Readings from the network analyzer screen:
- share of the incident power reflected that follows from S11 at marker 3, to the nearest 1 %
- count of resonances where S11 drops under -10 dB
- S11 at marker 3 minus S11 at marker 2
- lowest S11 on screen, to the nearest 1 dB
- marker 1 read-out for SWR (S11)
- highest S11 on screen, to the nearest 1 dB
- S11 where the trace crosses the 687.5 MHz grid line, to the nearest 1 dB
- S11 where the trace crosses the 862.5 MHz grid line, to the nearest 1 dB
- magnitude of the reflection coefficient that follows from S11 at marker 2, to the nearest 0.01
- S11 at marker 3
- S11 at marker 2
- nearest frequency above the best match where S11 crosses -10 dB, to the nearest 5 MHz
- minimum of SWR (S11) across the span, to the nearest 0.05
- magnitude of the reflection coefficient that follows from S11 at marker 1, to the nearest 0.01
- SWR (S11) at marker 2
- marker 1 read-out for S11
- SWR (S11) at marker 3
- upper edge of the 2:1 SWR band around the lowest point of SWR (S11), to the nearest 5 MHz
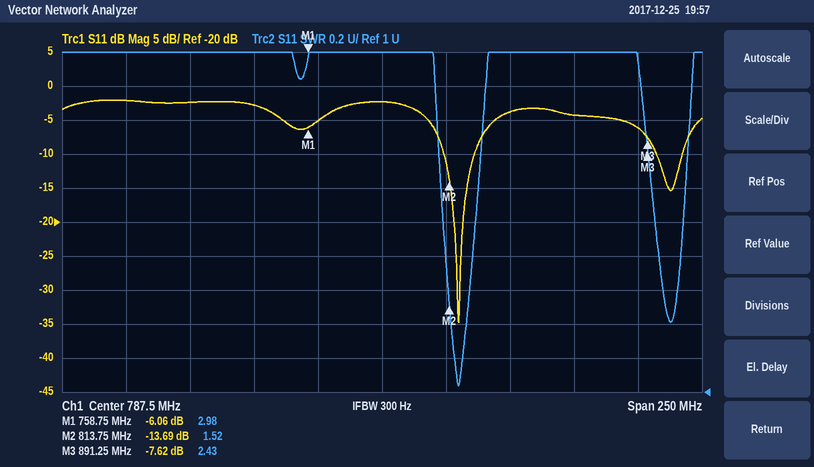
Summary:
17 %
2
6.07 dB
-35 dB
2.98
-2 dB
-2 dB
-4 dB
0.21
-7.62 dB
-13.69 dB
825 MHz
1.05
0.50
1.52
-6.06 dB
2.43
825 MHz
